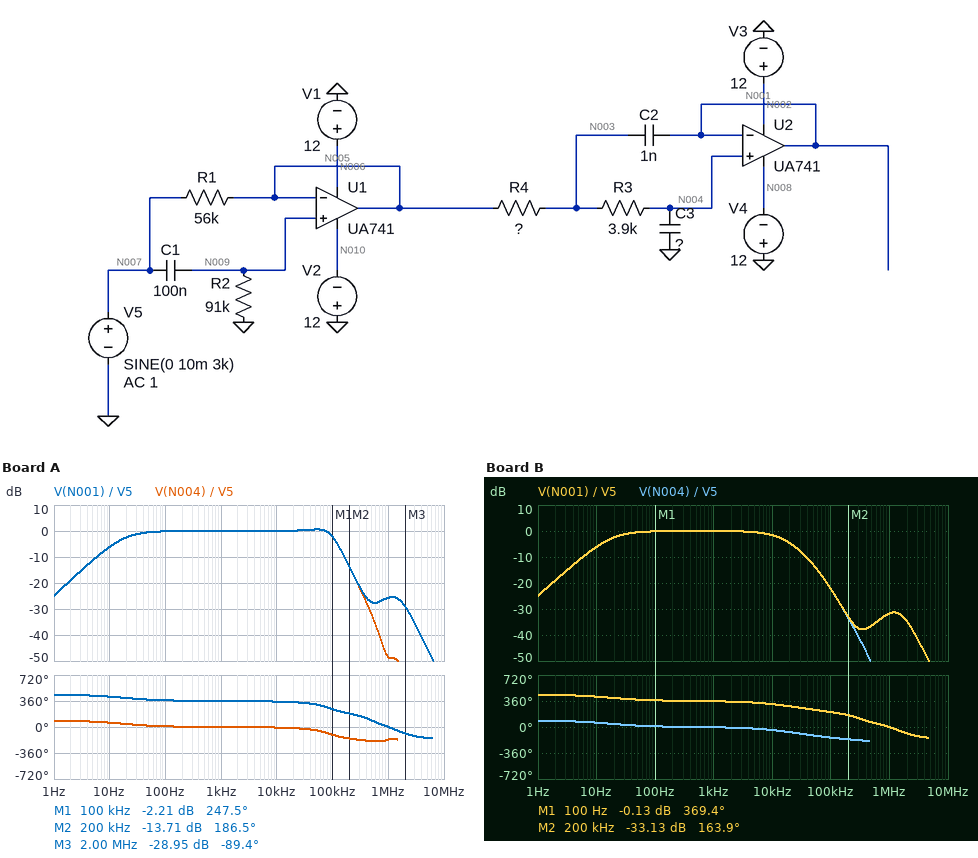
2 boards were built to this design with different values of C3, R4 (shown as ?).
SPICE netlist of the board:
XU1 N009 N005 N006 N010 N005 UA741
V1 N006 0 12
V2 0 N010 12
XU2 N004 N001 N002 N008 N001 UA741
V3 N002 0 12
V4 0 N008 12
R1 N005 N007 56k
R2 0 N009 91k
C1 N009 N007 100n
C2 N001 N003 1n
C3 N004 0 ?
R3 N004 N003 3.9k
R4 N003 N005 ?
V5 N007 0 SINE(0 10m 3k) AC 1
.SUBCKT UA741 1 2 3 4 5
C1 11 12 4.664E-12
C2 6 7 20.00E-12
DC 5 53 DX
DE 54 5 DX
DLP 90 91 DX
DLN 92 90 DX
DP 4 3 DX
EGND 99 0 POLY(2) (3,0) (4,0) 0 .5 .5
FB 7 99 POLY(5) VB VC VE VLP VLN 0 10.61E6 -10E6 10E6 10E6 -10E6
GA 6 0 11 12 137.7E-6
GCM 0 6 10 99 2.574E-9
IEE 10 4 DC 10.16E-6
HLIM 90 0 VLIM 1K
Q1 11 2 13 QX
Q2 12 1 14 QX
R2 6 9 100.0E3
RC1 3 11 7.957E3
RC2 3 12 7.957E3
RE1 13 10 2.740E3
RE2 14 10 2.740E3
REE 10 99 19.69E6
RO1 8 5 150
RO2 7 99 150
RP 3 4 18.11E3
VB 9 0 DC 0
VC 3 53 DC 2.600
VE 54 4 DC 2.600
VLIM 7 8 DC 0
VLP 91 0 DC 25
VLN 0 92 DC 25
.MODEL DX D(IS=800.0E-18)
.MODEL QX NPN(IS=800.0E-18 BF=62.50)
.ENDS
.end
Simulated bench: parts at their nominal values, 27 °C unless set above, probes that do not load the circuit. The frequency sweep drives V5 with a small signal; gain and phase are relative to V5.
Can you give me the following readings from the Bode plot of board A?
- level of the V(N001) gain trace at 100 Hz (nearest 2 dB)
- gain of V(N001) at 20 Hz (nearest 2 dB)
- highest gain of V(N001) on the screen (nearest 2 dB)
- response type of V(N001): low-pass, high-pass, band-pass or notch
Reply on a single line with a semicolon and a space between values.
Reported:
0 dB; -2 dB; 0 dB; band-pass
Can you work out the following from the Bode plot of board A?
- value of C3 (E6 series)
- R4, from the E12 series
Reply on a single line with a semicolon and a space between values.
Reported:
330 pF; 2.2 kΩ
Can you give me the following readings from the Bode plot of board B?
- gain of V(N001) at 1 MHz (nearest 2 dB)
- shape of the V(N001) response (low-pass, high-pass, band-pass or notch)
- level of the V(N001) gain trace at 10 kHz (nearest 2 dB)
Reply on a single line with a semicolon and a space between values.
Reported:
-32 dB; band-pass; -2 dB
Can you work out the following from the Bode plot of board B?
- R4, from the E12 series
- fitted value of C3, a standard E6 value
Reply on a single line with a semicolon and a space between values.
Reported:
4.7 kΩ; 1.5 nF
